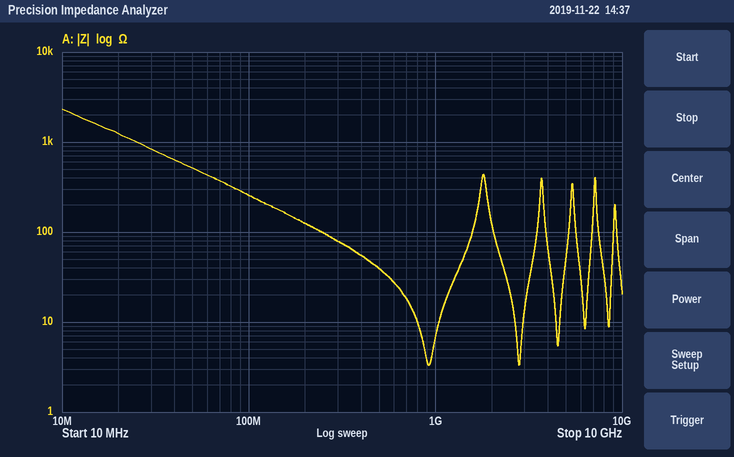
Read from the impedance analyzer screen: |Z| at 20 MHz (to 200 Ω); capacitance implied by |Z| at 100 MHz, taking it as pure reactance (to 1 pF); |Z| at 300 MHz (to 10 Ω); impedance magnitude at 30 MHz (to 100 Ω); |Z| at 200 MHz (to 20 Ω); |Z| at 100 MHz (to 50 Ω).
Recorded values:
1.2 kΩ
6 pF
80 Ω
800 Ω
120 Ω
250 Ω
